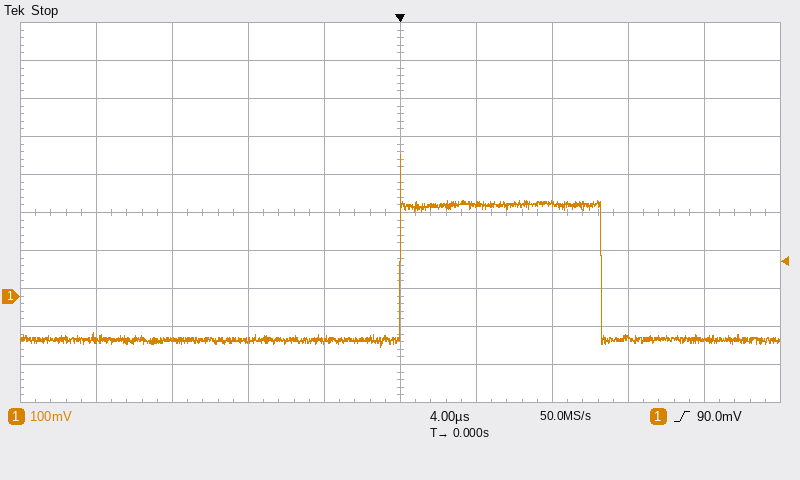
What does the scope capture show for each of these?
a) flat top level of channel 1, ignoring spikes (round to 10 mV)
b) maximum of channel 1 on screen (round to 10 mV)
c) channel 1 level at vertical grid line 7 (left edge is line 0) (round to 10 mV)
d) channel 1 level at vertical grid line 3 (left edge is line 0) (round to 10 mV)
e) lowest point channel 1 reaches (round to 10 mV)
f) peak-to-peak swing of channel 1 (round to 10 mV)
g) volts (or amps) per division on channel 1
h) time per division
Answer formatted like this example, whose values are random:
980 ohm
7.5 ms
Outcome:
240 mV
370 mV
240 mV
-120 mV
-140 mV
510 mV
100 mV
4 µs
